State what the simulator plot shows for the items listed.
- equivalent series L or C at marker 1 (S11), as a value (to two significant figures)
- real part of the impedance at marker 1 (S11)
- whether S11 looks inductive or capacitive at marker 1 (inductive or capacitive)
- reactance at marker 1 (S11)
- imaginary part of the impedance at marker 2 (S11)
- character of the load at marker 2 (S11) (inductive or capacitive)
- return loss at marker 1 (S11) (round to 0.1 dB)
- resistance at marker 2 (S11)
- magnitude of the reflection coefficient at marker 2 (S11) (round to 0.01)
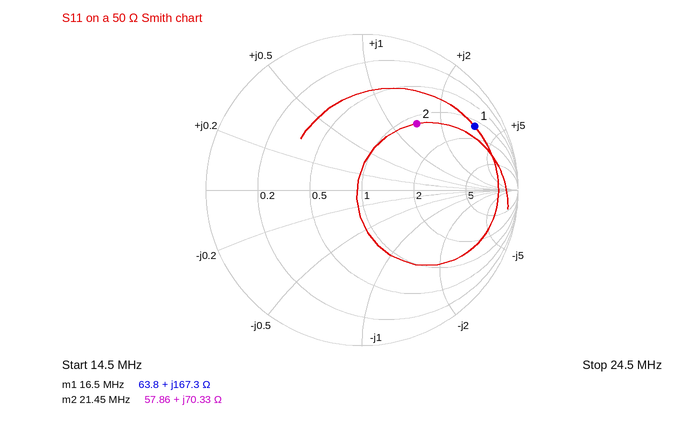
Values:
1.6 µH
63.8 Ω
inductive
+167.3 Ω
+70.33 Ω
inductive
1.6 dB
57.86 Ω
0.55
